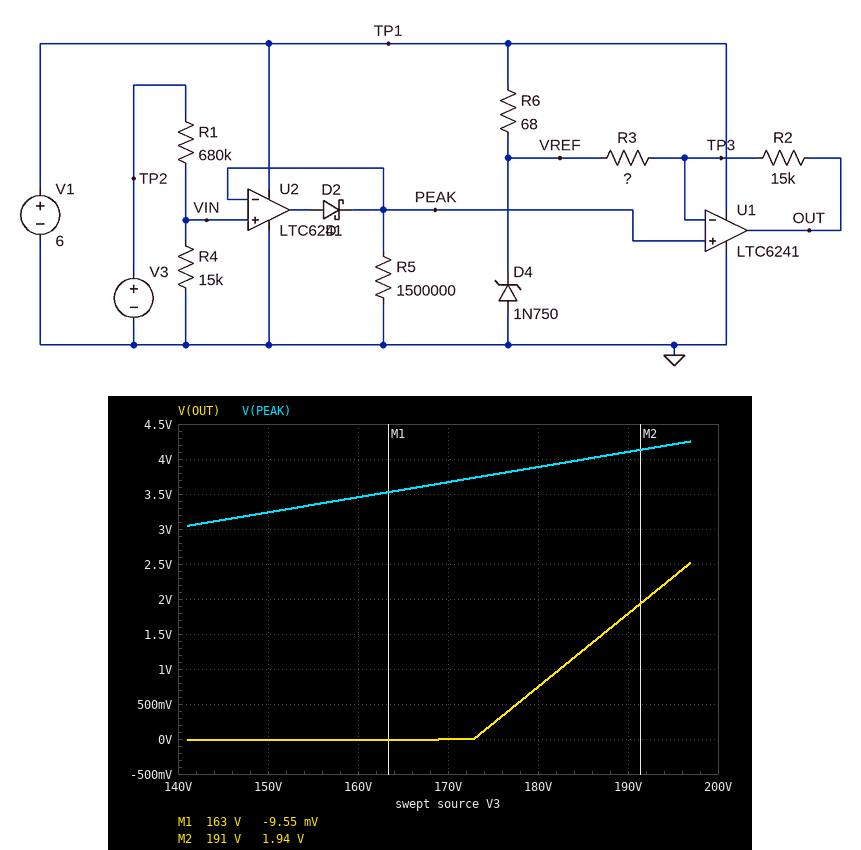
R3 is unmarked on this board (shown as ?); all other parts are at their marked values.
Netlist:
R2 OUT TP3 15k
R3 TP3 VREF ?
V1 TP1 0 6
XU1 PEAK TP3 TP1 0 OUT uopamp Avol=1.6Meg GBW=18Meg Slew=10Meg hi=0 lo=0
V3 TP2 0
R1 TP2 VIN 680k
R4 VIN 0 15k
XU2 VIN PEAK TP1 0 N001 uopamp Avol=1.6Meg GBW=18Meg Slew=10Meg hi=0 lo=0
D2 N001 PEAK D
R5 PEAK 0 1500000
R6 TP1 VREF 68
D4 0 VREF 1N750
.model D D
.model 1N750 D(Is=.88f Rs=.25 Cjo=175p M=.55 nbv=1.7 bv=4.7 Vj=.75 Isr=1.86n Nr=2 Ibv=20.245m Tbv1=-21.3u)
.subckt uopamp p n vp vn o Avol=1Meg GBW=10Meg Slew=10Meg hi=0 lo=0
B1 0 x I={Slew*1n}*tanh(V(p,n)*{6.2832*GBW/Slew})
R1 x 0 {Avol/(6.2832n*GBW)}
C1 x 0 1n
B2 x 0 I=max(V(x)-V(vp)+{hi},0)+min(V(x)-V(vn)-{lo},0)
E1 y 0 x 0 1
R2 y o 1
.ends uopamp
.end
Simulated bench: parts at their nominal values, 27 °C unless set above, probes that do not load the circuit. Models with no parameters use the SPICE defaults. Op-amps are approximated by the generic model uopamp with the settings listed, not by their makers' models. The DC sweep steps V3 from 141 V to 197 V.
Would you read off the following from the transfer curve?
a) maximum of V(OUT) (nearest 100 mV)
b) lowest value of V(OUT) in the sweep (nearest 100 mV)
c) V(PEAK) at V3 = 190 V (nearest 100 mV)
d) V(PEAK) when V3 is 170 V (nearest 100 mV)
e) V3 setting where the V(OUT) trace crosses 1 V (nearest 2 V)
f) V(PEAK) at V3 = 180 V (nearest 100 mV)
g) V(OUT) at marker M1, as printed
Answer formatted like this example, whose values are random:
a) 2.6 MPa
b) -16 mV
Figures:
a) 2.5 V
b) 0 V
c) 4.1 V
d) 3.7 V
e) 182 V
f) 3.9 V
g) -9.55 mV
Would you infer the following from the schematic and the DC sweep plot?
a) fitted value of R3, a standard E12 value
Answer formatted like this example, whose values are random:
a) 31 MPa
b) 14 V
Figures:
a) 3.9 kΩ
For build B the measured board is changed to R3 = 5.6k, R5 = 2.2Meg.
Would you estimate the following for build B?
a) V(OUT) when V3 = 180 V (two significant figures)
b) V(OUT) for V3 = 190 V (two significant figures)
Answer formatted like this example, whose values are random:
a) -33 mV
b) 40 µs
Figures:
a) 1.7 V
b) 2.5 V
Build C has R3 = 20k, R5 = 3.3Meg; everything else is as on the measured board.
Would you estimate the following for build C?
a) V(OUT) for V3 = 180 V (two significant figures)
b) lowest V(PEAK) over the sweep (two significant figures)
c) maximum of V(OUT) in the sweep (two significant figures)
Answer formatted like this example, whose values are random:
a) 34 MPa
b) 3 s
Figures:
a) 3.3 V
b) 3.0 V
c) 3.9 V
